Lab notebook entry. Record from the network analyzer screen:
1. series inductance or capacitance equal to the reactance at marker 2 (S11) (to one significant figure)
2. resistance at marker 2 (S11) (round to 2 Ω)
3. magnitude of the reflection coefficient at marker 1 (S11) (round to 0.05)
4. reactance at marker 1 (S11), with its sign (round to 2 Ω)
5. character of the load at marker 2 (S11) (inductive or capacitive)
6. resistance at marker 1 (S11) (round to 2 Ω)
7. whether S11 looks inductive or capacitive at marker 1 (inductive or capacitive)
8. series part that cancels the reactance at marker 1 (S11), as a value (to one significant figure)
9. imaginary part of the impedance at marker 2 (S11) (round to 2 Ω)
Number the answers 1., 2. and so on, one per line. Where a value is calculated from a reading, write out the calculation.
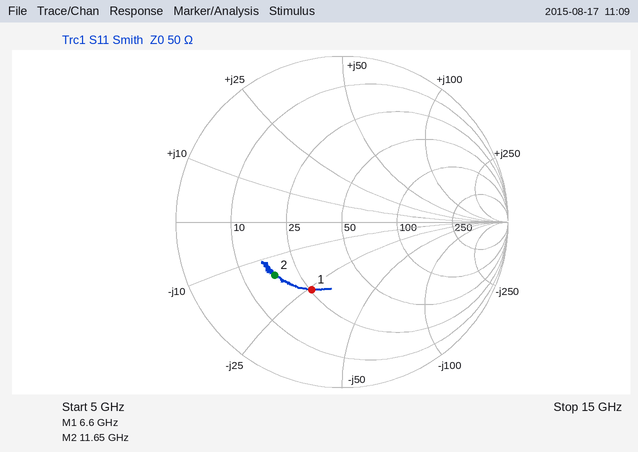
1. C = 1/(2π × 11.65 GHz × 16 Ω) ≈ 854 fF, so 900 fF to one significant figure
2. 18 Ω
3. 0.45
4. -26 Ω
5. capacitive
6. 26 Ω
7. capacitive
8. L = 26 Ω/(2π × 6.6 GHz) ≈ 627 pH, so 600 pH to one significant figure
9. -16 Ω
